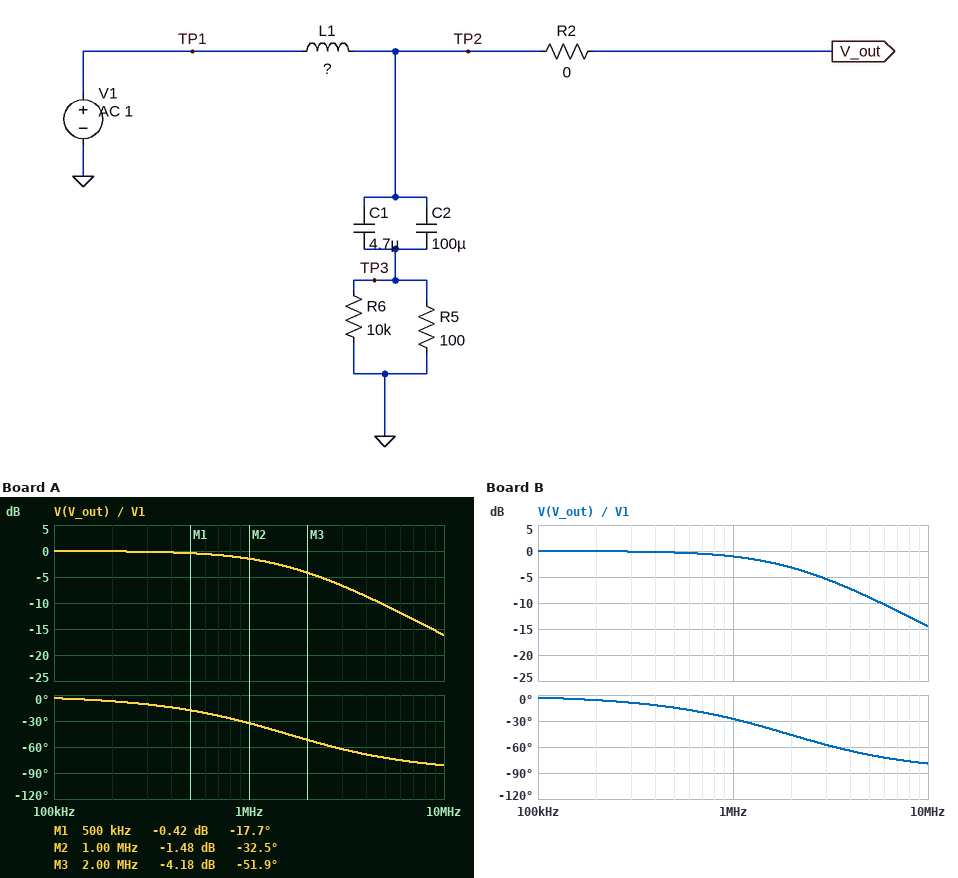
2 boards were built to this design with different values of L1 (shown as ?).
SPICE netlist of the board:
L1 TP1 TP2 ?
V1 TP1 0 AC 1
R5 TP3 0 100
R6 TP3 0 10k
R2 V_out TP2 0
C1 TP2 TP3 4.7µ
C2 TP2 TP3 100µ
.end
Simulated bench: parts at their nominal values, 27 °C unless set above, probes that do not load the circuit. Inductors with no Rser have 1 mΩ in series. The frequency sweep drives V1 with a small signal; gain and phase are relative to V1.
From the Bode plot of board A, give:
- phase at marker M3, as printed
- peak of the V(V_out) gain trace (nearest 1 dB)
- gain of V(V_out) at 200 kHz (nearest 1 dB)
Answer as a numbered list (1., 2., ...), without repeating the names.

1. -51.9 deg
2. 0 dB
3. 0 dB
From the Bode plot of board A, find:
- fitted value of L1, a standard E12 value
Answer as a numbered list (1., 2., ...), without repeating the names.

1. 10 µH
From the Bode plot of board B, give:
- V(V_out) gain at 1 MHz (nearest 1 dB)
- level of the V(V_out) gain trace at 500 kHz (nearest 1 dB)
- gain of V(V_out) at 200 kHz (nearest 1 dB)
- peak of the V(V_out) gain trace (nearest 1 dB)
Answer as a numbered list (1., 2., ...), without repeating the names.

1. -1 dB
2. 0 dB
3. 0 dB
4. 0 dB
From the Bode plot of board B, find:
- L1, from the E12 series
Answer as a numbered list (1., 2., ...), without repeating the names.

1. 8.2 µH
